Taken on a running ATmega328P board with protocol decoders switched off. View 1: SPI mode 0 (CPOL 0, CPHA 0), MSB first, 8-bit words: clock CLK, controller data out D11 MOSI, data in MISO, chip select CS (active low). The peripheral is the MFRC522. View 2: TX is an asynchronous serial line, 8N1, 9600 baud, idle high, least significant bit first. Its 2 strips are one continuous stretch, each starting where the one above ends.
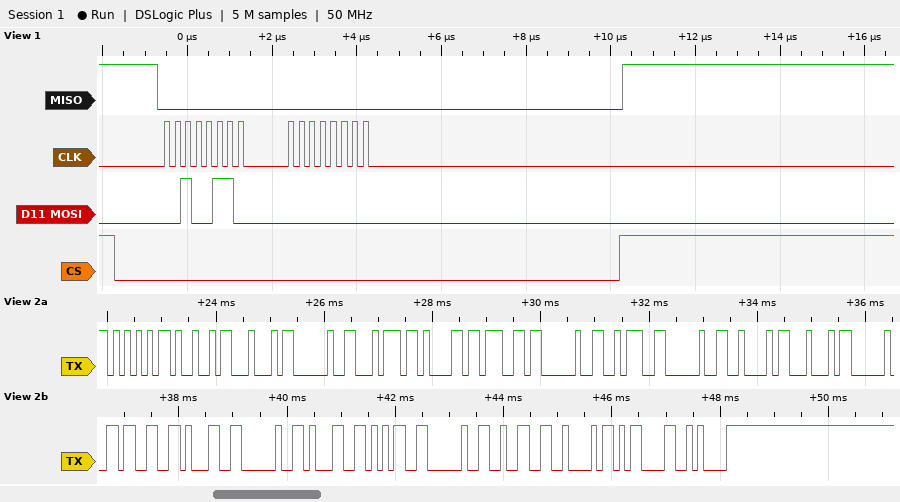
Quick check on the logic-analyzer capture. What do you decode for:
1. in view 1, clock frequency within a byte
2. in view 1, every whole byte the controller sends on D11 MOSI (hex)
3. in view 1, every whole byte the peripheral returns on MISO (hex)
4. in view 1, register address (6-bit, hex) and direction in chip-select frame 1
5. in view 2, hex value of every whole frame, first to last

4 MHz
26 00
00 00
0x13 write
0x55 0x49 0x44 0x20 0x74 0x61 0x67 0x20 0x3A 0x20 0x42 0x44 0x20 0x33 0x31 0x20 0x31 0x35 0x20 0x32 0x42 0x0D 0x0A
